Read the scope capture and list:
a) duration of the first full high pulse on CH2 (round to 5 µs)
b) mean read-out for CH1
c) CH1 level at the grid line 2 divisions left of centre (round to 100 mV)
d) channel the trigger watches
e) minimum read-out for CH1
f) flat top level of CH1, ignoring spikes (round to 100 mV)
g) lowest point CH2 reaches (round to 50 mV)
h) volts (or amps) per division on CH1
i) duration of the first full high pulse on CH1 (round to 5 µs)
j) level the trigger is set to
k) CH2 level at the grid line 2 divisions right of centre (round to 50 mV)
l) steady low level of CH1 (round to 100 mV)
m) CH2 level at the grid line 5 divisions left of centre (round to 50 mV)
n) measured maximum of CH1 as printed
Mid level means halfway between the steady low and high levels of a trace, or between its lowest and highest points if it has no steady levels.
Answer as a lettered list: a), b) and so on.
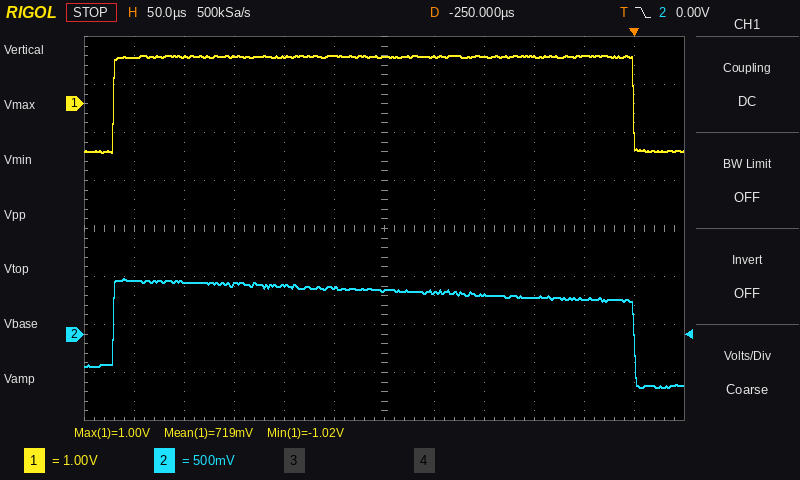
a) 520 µs
b) 719 mV
c) 1.0 V
d) CH2
e) -1.02 V
f) 1.0 V
g) -550 mV
h) 1 V
i) 520 µs
j) 0.00 V
k) 400 mV
l) -1.0 V
m) 550 mV
n) 1.00 V
